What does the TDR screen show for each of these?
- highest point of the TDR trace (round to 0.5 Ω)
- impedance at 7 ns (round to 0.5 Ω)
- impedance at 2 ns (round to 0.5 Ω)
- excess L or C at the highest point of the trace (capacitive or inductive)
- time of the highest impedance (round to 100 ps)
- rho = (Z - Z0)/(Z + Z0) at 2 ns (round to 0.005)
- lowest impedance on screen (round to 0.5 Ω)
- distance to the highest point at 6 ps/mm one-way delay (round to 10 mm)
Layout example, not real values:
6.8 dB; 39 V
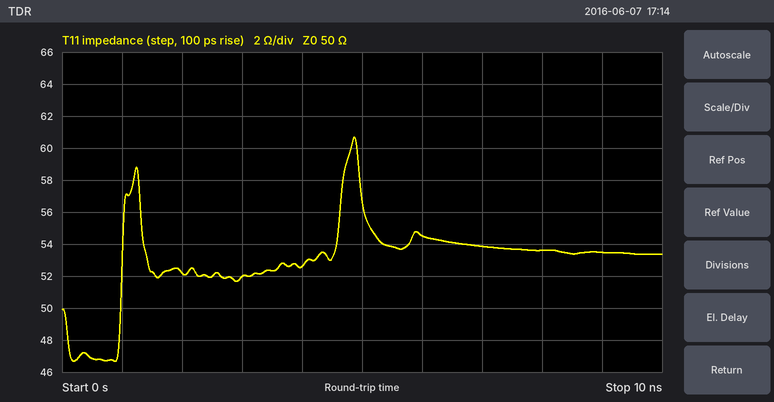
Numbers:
60.5 Ω; 54.0 Ω; 52.0 Ω; inductive; 4.9 ns; +0.020; 46.5 Ω; 410 mm
